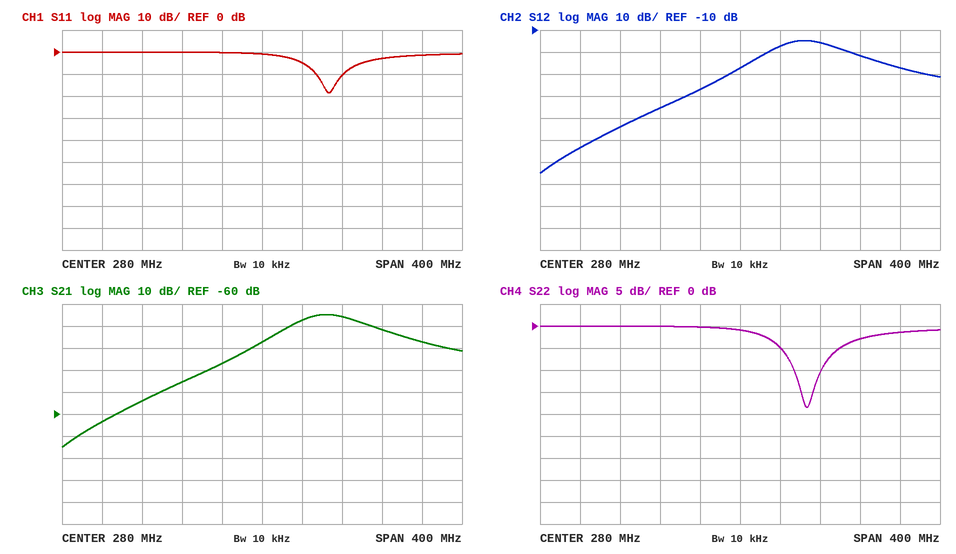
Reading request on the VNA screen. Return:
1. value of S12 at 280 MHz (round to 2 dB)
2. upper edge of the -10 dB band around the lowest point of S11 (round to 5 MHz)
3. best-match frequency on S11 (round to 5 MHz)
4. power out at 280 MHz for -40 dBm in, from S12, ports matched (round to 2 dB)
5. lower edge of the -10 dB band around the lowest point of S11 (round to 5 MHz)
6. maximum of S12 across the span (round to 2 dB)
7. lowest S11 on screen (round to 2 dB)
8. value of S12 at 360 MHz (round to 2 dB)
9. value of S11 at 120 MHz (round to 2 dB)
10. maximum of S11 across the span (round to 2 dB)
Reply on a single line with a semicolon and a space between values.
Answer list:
-28 dB; 360 MHz; 345 MHz; -68 dBm; 335 MHz; -14 dB; -18 dB; -16 dB; 0 dB; 0 dB
